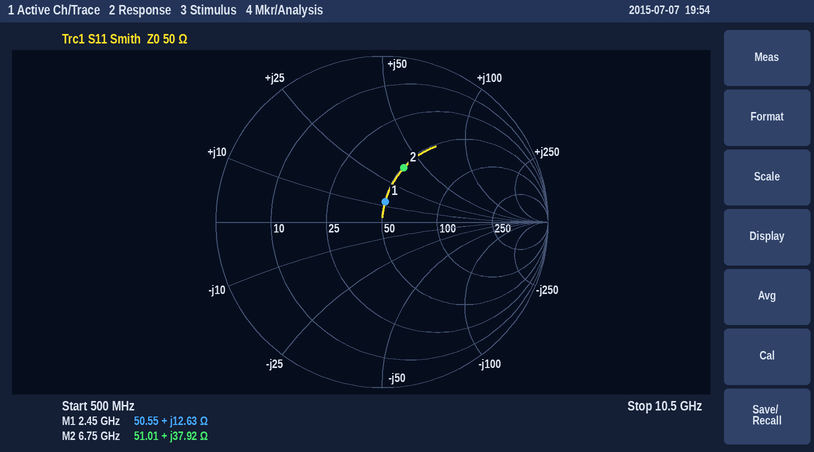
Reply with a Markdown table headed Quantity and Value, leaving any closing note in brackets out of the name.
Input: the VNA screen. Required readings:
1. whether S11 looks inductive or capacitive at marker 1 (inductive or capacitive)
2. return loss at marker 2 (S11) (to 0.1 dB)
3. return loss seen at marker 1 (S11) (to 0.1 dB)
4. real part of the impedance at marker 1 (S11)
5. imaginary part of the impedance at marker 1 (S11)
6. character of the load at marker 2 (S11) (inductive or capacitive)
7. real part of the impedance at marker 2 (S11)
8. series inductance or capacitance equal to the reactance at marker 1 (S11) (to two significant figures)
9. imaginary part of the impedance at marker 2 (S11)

| Quantity | Value |
|---|---|
| whether S11 looks inductive or capacitive at marker 1 | inductive |
| return loss at marker 2 (S11) | 9.1 dB |
| return loss seen at marker 1 (S11) | 18.1 dB |
| real part of the impedance at marker 1 | 50.55 Ω |
| imaginary part of the impedance at marker 1 | +12.63 Ω |
| character of the load at marker 2 (S11) | inductive |
| real part of the impedance at marker 2 | 51.01 Ω |
| series inductance or capacitance equal to the reactance at marker 1 (S11) | 820 pH |
| imaginary part of the impedance at marker 2 | +37.92 Ω |
